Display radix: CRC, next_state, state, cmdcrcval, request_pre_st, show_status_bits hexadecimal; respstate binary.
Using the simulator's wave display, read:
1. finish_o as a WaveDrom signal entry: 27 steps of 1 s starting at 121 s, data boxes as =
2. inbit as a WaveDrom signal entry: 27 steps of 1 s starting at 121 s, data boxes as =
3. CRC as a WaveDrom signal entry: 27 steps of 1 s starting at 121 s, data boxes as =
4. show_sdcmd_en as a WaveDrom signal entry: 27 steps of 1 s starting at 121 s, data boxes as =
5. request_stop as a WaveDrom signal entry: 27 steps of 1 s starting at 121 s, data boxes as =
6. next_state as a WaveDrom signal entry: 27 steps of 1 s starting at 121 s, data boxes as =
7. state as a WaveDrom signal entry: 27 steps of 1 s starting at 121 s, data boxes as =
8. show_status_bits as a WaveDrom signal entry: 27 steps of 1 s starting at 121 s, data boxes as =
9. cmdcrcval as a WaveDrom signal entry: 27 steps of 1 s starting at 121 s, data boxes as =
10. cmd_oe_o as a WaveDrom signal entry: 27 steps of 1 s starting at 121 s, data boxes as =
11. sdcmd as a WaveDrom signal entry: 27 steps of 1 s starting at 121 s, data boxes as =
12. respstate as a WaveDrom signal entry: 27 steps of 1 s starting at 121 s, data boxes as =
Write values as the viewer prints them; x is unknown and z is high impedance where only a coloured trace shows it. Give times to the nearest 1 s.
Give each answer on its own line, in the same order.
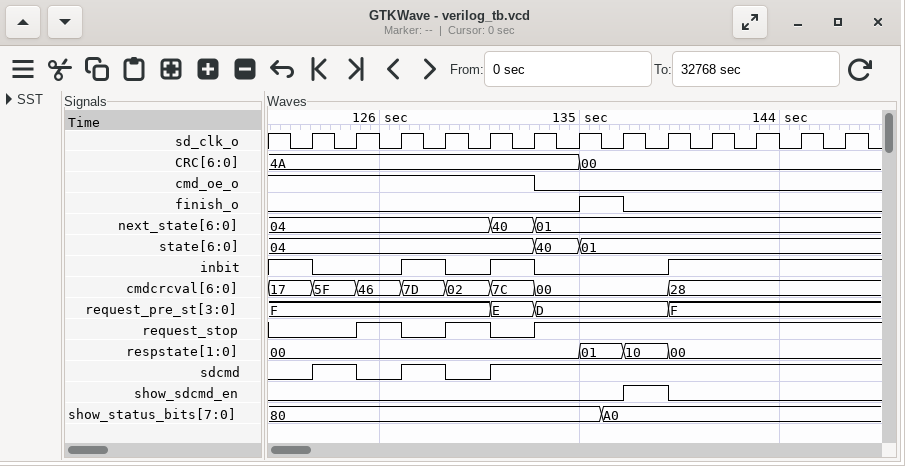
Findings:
{name: 'finish_o', wave: '0.............1.0..........'}
{name: 'inbit', wave: '1.0...1.0.1.0.....1........'}
{name: 'CRC', wave: '=.............=............', data: '4A 00'}
{name: 'show_sdcmd_en', wave: '0...............1.0........'}
{name: 'request_stop', wave: '0...1.0.1.0.1..............'}
{name: 'next_state', wave: '=.........=.=..............', data: '04 40 01'}
{name: 'state', wave: '=...........=.=............', data: '04 40 01'}
{name: 'show_status_bits', wave: '=..............=...........', data: '80 A0'}
{name: 'cmdcrcval', wave: '=.=.=.=.=.=.=.....=........', data: '17 5F 46 7D 02 7C 00 28'}
{name: 'cmd_oe_o', wave: '1...........0..............'}
{name: 'sdcmd', wave: '0.1.0.1.0.1................'}
{name: 'respstate', wave: '=.............=.=.=........', data: '00 01 10 00'}
